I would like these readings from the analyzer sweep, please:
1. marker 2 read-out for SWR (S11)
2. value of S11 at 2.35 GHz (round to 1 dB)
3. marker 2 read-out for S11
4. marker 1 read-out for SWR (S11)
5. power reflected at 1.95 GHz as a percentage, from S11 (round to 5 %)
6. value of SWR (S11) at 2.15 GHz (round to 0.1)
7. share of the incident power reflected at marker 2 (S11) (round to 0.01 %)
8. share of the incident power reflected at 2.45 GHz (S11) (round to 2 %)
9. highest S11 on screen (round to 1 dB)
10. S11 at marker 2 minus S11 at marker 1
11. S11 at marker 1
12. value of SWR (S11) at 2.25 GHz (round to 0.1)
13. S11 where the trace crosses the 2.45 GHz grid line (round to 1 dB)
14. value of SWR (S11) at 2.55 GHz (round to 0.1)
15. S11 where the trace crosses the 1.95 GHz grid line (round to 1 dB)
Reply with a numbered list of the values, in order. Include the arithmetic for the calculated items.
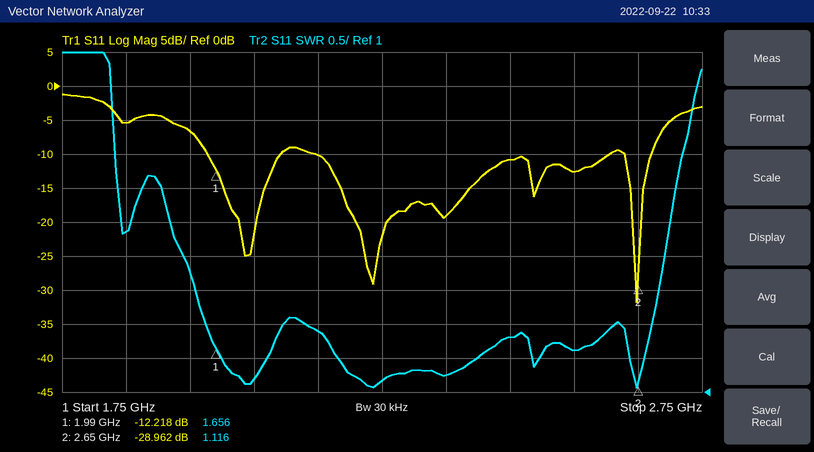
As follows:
1. 1.116
2. -19 dB
3. -28.962 dB
4. 1.656
5. 10^(-7/10) ≈ 20 %
6. 1.9
7. 10^(-28.962/10) ≈ 0.13 %
8. 10^(-11/10) ≈ 8 %
9. -1 dB
10. -28.962 − (-12.218) = -16.744 dB
11. -12.218 dB
12. 1.2
13. -11 dB
14. 1.6
15. -7 dB
